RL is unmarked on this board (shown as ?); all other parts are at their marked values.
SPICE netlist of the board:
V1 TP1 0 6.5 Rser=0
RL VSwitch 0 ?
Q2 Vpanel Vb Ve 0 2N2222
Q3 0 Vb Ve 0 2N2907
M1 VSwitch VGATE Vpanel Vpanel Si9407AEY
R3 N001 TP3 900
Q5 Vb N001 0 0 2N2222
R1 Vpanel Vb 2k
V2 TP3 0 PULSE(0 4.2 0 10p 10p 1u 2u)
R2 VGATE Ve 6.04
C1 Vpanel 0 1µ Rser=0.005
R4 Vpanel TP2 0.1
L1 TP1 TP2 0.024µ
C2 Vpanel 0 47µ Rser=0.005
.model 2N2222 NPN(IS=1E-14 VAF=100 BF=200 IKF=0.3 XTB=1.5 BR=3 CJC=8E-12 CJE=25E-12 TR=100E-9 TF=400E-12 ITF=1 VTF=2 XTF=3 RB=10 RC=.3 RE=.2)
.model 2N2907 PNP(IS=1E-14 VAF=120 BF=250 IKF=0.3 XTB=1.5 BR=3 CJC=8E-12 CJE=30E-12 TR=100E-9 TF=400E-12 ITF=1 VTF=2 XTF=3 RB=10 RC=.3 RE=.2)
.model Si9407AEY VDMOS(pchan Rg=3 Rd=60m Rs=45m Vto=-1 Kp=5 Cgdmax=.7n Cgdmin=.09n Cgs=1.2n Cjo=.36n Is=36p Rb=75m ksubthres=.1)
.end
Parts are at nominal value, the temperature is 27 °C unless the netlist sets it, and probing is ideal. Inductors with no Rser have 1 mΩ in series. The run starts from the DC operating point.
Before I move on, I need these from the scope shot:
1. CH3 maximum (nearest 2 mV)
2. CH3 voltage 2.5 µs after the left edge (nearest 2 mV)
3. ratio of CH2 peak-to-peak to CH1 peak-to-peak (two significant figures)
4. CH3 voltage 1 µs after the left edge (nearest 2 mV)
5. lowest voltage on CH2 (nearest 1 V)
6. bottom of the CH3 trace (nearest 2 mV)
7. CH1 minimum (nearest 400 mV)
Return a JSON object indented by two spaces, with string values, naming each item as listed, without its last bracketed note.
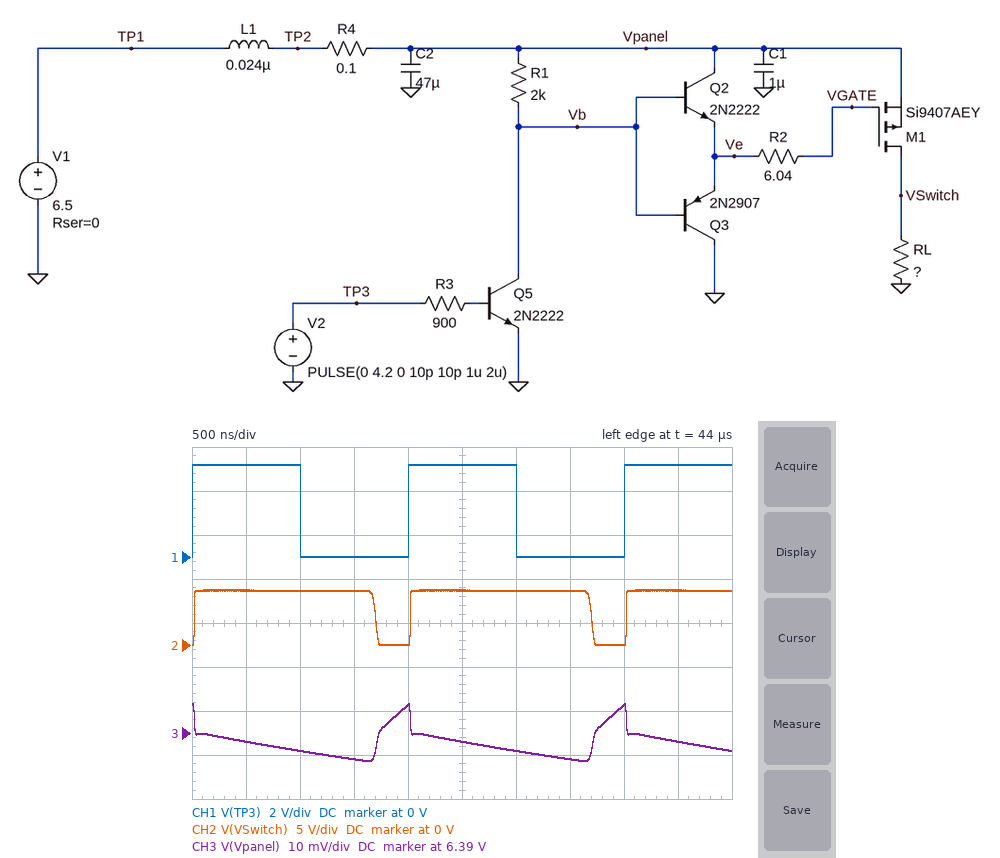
{
  "CH3 maximum": "6.396 V",
  "CH3 voltage 2.5 µs after the left edge": "6.388 V",
  "ratio of CH2 peak-to-peak to CH1 peak-to-peak": "1.5",
  "CH3 voltage 1 µs after the left edge": "6.386 V",
  "lowest voltage on CH2": "0 V",
  "bottom of the CH3 trace": "6.384 V",
  "CH1 minimum": "0 V"
}
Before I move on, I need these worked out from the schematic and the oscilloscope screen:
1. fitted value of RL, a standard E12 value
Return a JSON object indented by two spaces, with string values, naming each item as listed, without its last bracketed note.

{
  "fitted value of RL, a standard E12 value": "4.7 Ω"
}
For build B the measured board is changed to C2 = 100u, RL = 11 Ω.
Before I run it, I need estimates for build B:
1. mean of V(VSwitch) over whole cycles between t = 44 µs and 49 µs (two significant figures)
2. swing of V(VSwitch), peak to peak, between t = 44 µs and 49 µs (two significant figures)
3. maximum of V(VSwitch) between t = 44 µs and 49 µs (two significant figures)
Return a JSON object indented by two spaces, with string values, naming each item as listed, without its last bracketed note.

{
  "mean of V(VSwitch) over whole cycles between t = 44 µs and 49 µs": "5.4 V",
  "swing of V(VSwitch), peak to peak, between t = 44 µs and 49 µs": "6.5 V",
  "maximum of V(VSwitch) between t = 44 µs and 49 µs": "6.4 V"
}
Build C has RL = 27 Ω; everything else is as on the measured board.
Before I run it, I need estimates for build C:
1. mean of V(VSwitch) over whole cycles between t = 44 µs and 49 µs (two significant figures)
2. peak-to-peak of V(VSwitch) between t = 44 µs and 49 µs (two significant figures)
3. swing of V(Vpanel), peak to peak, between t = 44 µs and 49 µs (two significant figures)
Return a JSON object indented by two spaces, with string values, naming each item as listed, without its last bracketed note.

{
  "mean of V(VSwitch) over whole cycles between t = 44 µs and 49 µs": "5.5 V",
  "peak-to-peak of V(VSwitch) between t = 44 µs and 49 µs": "6.6 V",
  "swing of V(Vpanel), peak to peak, between t = 44 µs and 49 µs": "2.5 mV"
}
